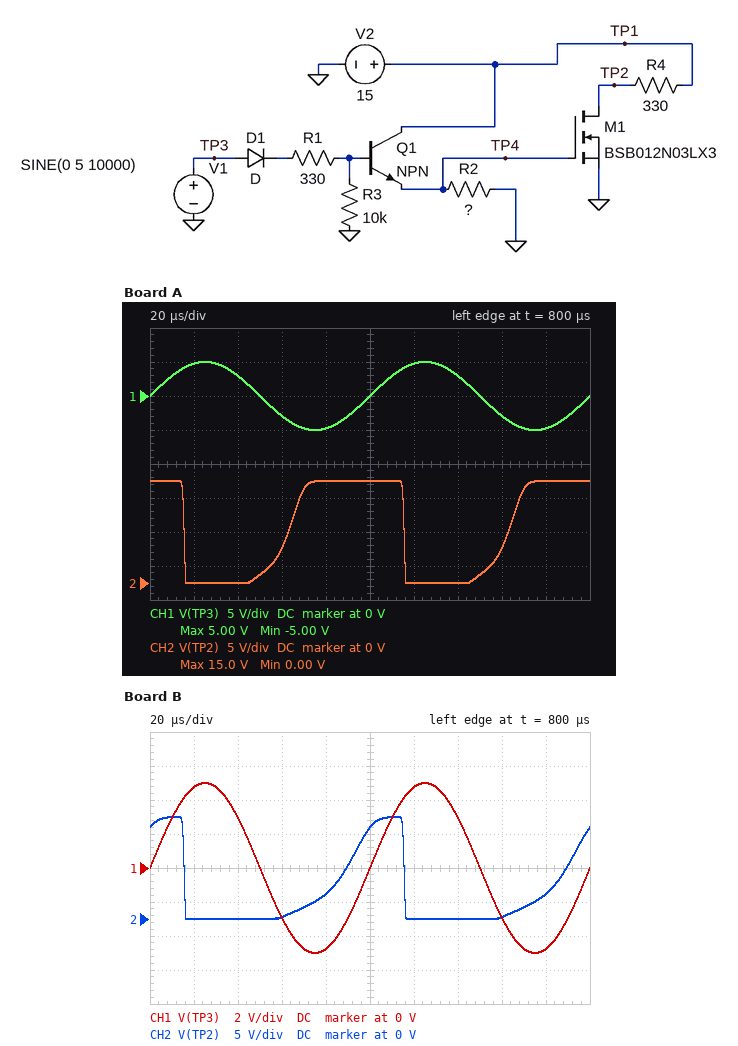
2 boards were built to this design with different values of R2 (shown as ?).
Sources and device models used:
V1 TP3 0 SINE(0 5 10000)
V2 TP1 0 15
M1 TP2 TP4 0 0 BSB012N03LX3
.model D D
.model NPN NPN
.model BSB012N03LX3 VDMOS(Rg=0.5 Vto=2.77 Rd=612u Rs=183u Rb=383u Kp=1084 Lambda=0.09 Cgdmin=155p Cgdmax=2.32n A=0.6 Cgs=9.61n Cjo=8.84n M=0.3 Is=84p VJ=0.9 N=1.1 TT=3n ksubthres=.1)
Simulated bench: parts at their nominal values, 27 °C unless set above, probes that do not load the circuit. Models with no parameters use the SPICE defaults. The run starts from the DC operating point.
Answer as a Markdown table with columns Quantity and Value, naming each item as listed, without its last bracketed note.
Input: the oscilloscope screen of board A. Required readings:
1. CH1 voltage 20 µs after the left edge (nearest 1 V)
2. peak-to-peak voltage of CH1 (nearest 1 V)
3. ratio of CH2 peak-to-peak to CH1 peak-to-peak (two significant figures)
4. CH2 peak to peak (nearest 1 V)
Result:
| Quantity | Value |
|---|---|
| CH1 voltage 20 µs after the left edge | 5 V |
| peak-to-peak voltage of CH1 | 10 V |
| ratio of CH2 peak-to-peak to CH1 peak-to-peak | 1.5 |
| CH2 peak to peak | 15 V |
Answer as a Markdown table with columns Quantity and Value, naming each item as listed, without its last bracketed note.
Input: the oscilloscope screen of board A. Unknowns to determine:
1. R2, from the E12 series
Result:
| Quantity | Value |
|---|---|
| R2, from the E12 series | 4.7 kΩ |
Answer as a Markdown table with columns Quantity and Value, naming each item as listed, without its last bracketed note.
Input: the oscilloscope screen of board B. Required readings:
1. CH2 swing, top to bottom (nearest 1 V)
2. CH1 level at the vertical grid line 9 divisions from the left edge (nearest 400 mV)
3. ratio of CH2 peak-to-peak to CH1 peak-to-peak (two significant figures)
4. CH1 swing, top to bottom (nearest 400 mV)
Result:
| Quantity | Value |
|---|---|
| CH2 swing, top to bottom | 15 V |
| CH1 level at the vertical grid line 9 divisions from the left edge | -4.8 V |
| ratio of CH2 peak-to-peak to CH1 peak-to-peak | 1.5 |
| CH1 swing, top to bottom | 10.0 V |
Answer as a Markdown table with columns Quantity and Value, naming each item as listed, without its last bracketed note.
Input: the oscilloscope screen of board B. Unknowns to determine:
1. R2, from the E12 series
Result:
| Quantity | Value |
|---|---|
| R2, from the E12 series | 8.2 kΩ |
